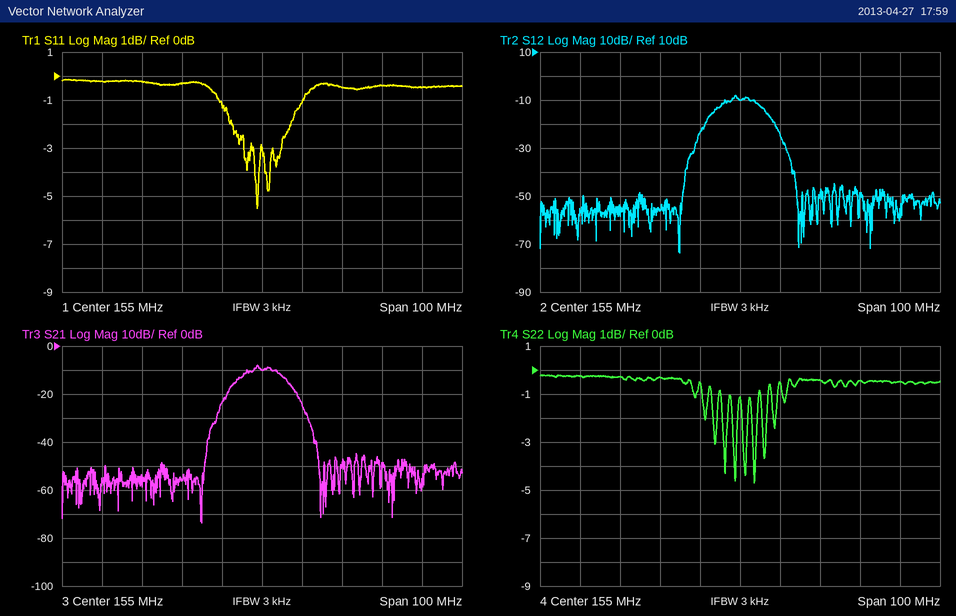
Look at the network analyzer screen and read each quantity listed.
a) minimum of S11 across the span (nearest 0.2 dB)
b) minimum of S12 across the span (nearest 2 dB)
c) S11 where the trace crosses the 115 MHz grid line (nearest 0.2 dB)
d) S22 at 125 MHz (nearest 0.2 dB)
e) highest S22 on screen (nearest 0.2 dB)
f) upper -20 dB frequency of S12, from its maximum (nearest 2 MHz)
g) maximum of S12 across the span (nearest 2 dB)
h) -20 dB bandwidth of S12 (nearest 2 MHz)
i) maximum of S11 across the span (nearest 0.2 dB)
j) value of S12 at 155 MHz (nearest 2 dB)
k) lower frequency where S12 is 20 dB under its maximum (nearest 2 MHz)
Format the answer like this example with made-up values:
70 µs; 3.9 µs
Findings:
-5.6 dB; -74 dB; -0.2 dB; -0.2 dB; -0.2 dB; 166 MHz; -8 dB; 22 MHz; -0.2 dB; -10 dB; 144 MHz
